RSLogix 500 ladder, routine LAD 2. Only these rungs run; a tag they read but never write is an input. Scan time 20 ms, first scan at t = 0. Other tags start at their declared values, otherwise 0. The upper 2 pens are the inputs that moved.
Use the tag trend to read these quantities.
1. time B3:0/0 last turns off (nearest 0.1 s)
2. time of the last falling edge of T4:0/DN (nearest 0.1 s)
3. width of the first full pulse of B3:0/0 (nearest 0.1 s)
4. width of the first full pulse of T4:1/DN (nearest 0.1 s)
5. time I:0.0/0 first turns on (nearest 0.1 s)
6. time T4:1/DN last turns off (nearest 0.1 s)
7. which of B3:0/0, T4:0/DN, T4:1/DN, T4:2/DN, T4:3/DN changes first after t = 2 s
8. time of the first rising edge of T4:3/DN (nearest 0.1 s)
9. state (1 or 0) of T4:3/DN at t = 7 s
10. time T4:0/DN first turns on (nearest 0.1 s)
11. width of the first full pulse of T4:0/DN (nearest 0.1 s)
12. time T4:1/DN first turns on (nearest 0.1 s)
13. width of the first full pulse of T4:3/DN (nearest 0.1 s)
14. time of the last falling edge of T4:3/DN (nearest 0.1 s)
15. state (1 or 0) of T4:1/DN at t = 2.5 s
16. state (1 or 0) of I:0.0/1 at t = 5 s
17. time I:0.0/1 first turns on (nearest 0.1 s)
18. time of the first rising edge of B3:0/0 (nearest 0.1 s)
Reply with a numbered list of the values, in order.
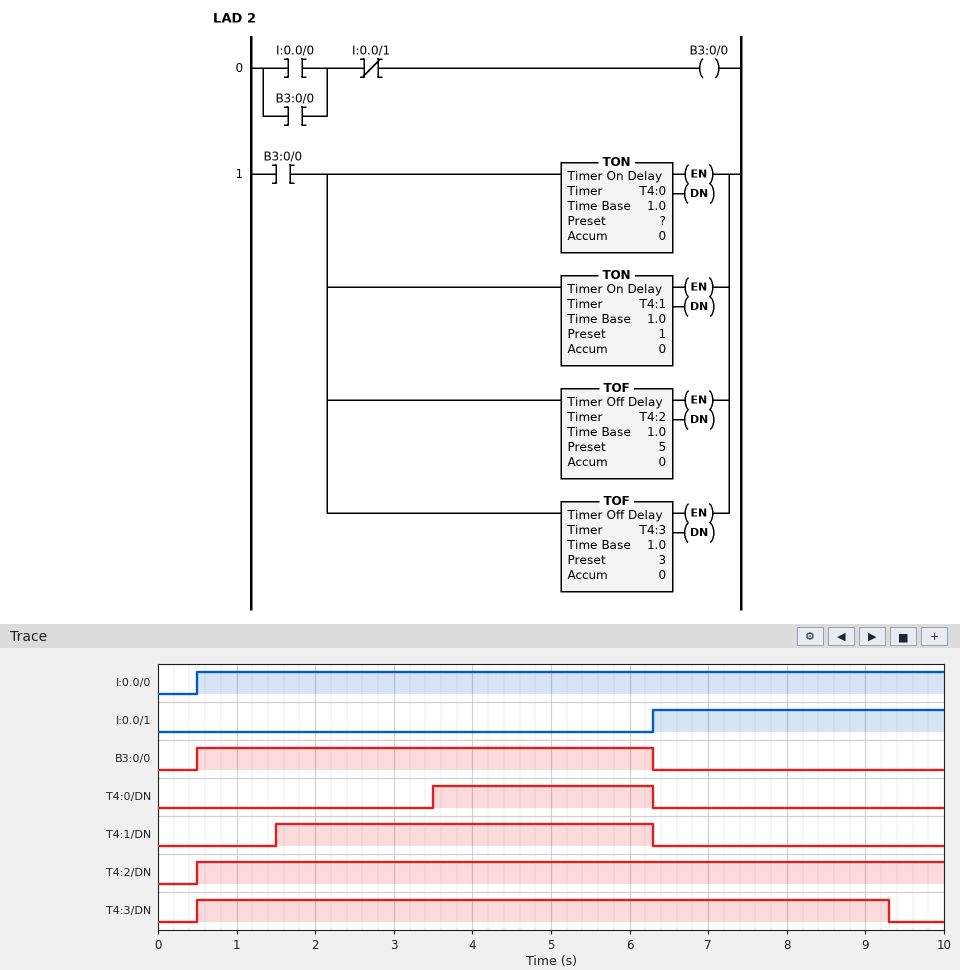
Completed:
1. 6.3 s
2. 6.3 s
3. 5.8 s
4. 4.8 s
5. 0.5 s
6. 6.3 s
7. T4:0/DN
8. 0.5 s
9. 1
10. 3.5 s
11. 2.8 s
12. 1.5 s
13. 8.8 s
14. 9.3 s
15. 1
16. 0
17. 6.3 s
18. 0.5 s
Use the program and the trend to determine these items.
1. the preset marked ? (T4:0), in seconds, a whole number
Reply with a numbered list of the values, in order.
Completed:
1. 3 s
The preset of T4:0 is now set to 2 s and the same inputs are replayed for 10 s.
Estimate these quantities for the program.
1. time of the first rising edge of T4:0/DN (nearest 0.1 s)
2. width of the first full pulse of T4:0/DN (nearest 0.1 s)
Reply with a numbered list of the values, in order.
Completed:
1. 2.5 s
2. 3.8 s
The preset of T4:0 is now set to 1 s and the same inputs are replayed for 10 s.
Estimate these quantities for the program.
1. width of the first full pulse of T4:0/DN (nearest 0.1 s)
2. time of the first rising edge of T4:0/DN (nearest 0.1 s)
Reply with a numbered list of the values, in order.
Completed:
1. 4.8 s
2. 1.5 s
